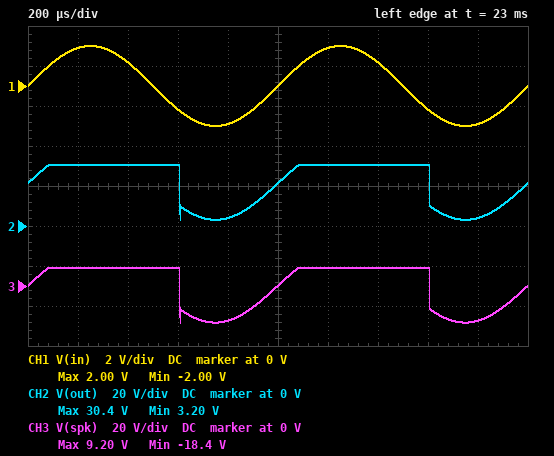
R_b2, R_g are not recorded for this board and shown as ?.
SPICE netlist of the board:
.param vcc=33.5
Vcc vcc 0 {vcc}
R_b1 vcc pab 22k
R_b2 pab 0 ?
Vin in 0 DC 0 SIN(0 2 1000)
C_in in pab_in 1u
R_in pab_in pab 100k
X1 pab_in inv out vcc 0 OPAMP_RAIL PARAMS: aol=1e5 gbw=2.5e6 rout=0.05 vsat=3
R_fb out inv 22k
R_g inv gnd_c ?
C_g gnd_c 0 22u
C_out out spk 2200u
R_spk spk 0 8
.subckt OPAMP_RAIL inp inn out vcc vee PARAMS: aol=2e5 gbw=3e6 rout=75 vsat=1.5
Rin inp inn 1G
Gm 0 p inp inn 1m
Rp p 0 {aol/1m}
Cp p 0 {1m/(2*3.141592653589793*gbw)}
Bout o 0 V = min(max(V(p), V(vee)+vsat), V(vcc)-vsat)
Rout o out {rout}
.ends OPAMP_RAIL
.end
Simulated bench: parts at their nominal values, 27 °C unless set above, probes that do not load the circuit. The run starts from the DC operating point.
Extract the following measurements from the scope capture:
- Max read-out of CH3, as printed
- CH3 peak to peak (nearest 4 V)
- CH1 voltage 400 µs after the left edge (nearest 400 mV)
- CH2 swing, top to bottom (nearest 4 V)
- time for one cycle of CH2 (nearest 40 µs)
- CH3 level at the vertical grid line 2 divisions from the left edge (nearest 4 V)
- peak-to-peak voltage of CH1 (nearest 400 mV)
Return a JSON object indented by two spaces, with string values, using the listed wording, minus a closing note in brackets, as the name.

{
  "Max read-out of CH3, as printed": "9.20 V",
  "CH3 peak to peak": "28 V",
  "CH1 voltage 400 µs after the left edge": "1.2 V",
  "CH2 swing, top to bottom": "28 V",
  "time for one cycle of CH2": "1.00 ms",
  "CH3 level at the vertical grid line 2 divisions from the left edge": "8 V",
  "peak-to-peak voltage of CH1": "4.0 V"
}
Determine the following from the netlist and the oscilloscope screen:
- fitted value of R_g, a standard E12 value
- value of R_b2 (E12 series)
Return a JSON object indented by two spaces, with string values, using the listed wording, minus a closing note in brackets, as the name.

{
  "fitted value of R_g, a standard E12 value": "2.7 kΩ",
  "value of R_b2": "39 kΩ"
}
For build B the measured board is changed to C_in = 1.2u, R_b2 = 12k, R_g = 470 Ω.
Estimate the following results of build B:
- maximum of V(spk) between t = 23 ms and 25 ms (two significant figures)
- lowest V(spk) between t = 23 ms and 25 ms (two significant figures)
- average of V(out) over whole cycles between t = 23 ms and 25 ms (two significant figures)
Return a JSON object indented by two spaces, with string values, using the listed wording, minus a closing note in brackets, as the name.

{
  "maximum of V(spk) between t = 23 ms and 25 ms": "19 V",
  "lowest V(spk) between t = 23 ms and 25 ms": "-9.1 V",
  "average of V(out) over whole cycles between t = 23 ms and 25 ms": "12 V"
}
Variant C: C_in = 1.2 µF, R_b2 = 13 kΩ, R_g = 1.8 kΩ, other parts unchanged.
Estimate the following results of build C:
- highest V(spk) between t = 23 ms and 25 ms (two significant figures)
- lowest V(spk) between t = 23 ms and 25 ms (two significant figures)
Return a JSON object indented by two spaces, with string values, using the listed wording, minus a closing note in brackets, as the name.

{
  "highest V(spk) between t = 23 ms and 25 ms": "18 V",
  "lowest V(spk) between t = 23 ms and 25 ms": "-9.6 V"
}
